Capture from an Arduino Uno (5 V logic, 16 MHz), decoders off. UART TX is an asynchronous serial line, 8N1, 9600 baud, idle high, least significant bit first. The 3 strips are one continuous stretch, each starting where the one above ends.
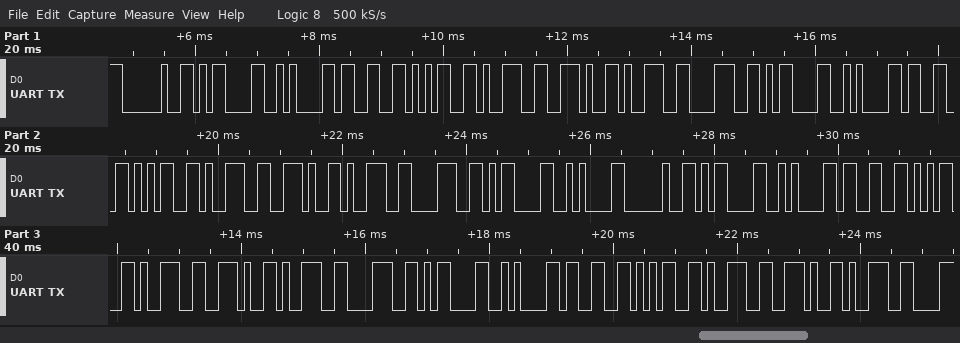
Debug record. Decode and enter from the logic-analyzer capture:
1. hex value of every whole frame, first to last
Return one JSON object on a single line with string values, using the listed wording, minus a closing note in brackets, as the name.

{"hex value of every whole frame, first to last": "20 0D 0A 33 35 39 2E 39 38 0D 0A 33 35 39 2E 39 38 0D 0A 20 0D 0A 33 35 39 2E 39 38 0D 0A 33 35 39 2E 39"}
